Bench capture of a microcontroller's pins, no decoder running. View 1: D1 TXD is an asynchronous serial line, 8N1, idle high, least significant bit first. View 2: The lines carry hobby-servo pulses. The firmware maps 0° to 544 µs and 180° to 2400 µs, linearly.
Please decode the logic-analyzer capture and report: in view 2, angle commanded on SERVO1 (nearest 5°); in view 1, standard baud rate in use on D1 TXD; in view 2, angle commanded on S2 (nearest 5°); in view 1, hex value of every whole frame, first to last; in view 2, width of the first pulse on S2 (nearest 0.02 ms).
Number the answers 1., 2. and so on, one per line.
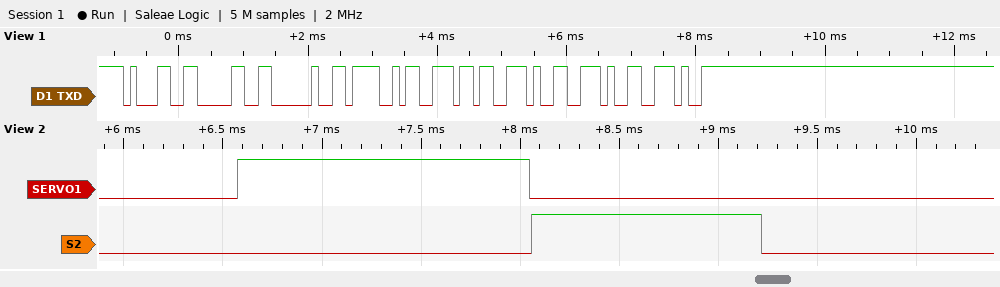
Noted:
1. 90°
2. 9600 baud
3. 60°
4. 31 30 20 4F 6E 2E 2E 2E
5. 1.16 ms
